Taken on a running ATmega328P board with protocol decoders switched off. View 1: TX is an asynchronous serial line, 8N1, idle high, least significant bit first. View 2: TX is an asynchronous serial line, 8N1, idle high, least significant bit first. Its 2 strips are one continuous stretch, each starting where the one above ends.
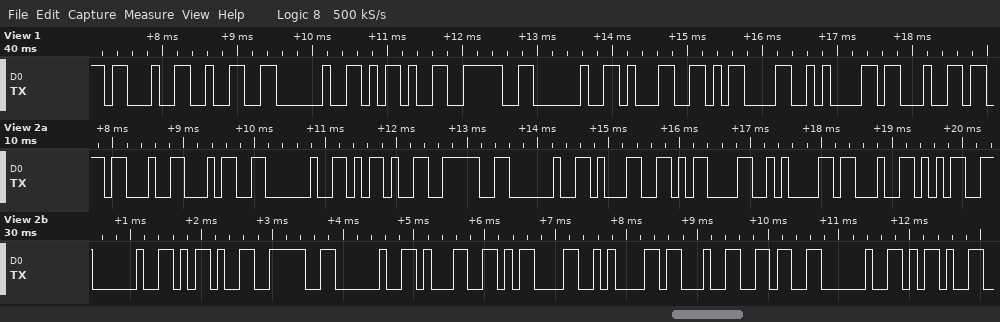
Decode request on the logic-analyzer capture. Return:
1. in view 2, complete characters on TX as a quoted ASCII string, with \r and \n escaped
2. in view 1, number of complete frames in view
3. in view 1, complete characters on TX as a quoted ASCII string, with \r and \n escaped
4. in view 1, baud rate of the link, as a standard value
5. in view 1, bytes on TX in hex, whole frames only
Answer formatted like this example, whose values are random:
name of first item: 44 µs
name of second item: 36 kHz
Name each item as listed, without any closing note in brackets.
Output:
in view 2, complete characters on TX as a quoted ASCII string, with \r and \n escaped: "#4 -> 1\r\n#5 -> 1\r\n#6 -"
in view 1, number of complete frames in view: 10
in view 1, complete characters on TX as a quoted ASCII string, with \r and \n escaped: "#2 -> 1\r\n#"
in view 1, baud rate of the link, as a standard value: 9600 baud
in view 1, bytes on TX in hex, whole frames only: 23 32 20 2D 3E 20 31 0D 0A 23
